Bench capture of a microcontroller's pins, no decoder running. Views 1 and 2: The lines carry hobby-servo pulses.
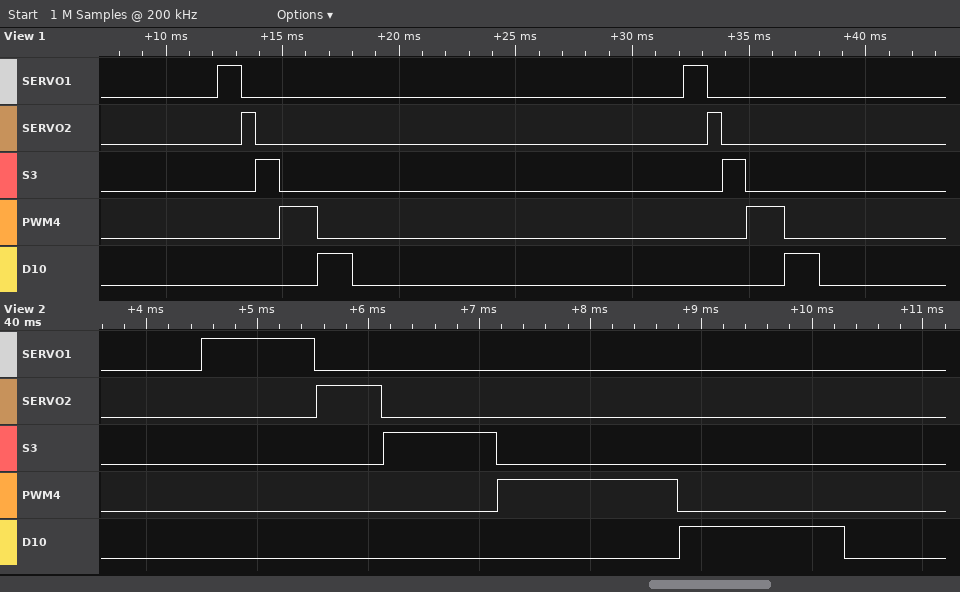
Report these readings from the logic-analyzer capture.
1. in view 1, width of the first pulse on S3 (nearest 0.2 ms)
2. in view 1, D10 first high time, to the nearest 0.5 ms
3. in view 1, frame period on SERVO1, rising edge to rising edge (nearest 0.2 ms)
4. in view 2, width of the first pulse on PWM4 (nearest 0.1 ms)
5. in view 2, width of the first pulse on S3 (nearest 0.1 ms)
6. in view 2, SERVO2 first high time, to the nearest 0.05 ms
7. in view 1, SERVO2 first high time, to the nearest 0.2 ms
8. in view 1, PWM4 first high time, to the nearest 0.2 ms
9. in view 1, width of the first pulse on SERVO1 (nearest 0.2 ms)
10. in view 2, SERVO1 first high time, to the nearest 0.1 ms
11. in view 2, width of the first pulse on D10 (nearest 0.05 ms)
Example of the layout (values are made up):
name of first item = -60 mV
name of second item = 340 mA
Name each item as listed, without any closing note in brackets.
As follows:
in view 1, width of the first pulse on S3 = 1.0 ms
in view 1, D10 first high time, to the nearest 0.5 ms = 1.5 ms
in view 1, frame period on SERVO1, rising edge to rising edge = 20.0 ms
in view 2, width of the first pulse on PWM4 = 1.6 ms
in view 2, width of the first pulse on S3 = 1.0 ms
in view 2, SERVO2 first high time, to the nearest 0.05 ms = 0.60 ms
in view 1, SERVO2 first high time, to the nearest 0.2 ms = 0.6 ms
in view 1, PWM4 first high time, to the nearest 0.2 ms = 1.6 ms
in view 1, width of the first pulse on SERVO1 = 1.0 ms
in view 2, SERVO1 first high time, to the nearest 0.1 ms = 1.0 ms
in view 2, width of the first pulse on D10 = 1.50 ms
